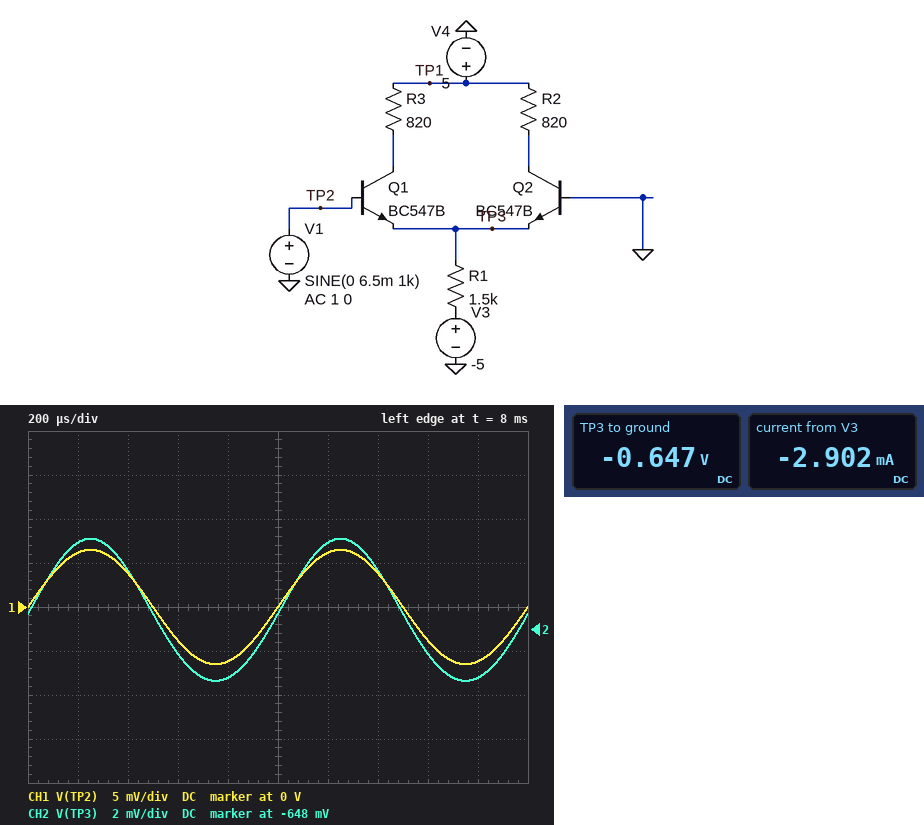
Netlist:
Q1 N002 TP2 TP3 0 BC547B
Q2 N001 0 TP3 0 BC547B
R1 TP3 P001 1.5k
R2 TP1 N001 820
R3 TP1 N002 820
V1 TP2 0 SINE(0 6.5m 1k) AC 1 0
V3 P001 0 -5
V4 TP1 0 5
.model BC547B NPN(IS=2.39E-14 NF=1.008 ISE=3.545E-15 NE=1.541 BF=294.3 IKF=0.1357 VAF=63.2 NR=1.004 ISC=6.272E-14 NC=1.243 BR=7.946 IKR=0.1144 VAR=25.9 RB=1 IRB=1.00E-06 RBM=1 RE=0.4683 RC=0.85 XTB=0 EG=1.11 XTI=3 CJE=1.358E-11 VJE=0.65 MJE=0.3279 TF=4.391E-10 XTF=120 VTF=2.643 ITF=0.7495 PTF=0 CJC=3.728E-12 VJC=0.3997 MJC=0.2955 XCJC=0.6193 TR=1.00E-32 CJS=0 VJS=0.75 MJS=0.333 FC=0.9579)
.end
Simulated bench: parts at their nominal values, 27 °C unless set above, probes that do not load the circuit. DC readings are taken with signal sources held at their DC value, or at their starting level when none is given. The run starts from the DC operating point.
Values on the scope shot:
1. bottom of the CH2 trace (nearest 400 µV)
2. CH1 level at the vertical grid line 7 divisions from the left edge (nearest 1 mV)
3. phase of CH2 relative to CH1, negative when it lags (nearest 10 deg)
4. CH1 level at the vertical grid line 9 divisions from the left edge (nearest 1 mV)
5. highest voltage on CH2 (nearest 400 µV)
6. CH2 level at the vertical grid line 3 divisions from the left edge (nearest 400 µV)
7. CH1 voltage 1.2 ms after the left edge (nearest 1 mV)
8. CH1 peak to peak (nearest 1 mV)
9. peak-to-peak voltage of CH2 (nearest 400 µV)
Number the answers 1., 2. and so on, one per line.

1. -650.4 mV
2. 4 mV
3. 0 deg
4. -6 mV
5. -644.0 mV
6. -649.2 mV
7. 6 mV
8. 13 mV
9. 6.4 mV
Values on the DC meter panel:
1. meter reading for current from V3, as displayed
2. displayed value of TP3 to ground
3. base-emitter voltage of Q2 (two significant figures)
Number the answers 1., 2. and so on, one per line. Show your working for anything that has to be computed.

1. -2.902 mA
2. -0.647 V
3. 0 V - (-647 mV) = 650 mV
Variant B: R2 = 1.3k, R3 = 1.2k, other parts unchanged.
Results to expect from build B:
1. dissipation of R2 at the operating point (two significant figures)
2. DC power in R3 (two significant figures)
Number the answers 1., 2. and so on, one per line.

1. 2.7 mW
2. 2.5 mW
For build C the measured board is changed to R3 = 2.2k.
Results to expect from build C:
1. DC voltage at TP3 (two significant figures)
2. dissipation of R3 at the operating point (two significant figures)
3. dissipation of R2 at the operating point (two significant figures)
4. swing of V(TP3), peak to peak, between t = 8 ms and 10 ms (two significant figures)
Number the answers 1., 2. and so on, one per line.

1. -650 mV
2. 4.5 mW
3. 1.8 mW
4. 6.3 mV
